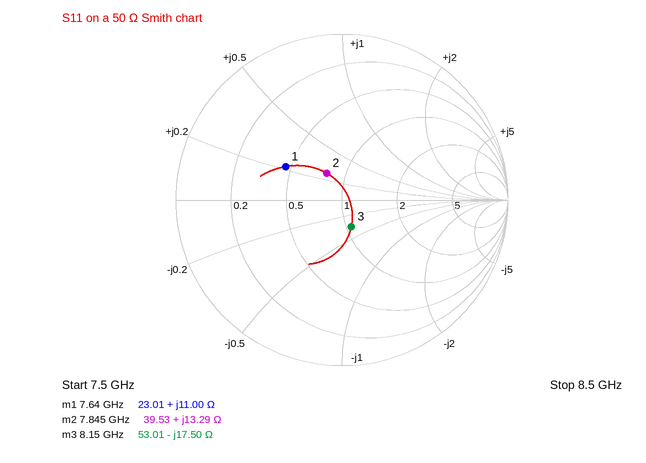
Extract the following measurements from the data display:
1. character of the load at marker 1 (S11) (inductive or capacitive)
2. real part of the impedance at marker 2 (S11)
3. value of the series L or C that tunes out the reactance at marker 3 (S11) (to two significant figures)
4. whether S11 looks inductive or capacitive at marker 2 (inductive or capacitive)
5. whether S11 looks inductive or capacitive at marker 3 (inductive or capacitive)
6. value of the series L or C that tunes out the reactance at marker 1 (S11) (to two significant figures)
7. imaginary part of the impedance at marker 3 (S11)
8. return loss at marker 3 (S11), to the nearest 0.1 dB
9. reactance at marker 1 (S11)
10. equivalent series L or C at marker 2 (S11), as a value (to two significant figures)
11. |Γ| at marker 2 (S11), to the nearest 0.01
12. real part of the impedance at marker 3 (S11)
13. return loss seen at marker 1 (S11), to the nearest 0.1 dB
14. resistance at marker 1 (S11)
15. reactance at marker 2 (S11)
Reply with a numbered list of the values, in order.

1. inductive
2. 39.53 Ω
3. 340 pH
4. inductive
5. capacitive
6. 1.9 pF
7. -17.50 Ω
8. 15.4 dB
9. +11.00 Ω
10. 270 pH
11. 0.19
12. 53.01 Ω
13. 8.1 dB
14. 23.01 Ω
15. +13.29 Ω
